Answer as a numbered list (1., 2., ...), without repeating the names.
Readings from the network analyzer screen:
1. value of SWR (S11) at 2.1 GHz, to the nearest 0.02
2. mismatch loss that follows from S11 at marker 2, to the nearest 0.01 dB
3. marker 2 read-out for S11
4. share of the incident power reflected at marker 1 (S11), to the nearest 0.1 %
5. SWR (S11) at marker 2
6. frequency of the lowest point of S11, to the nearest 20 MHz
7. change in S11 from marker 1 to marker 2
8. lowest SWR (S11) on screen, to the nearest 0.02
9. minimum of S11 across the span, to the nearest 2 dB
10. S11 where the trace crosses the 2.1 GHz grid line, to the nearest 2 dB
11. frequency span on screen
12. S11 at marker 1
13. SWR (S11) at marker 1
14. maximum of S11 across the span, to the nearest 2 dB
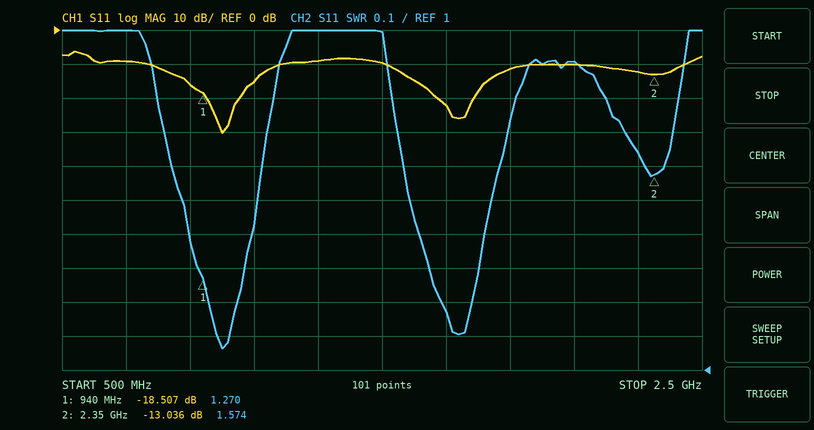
1. 1.90
2. 0.22 dB
3. -13.036 dB
4. 1.4 %
5. 1.574
6. 1.00 GHz
7. 5.471 dB
8. 1.06
9. -30 dB
10. -10 dB
11. 2 GHz
12. -18.507 dB
13. 1.270
14. -6 dB
